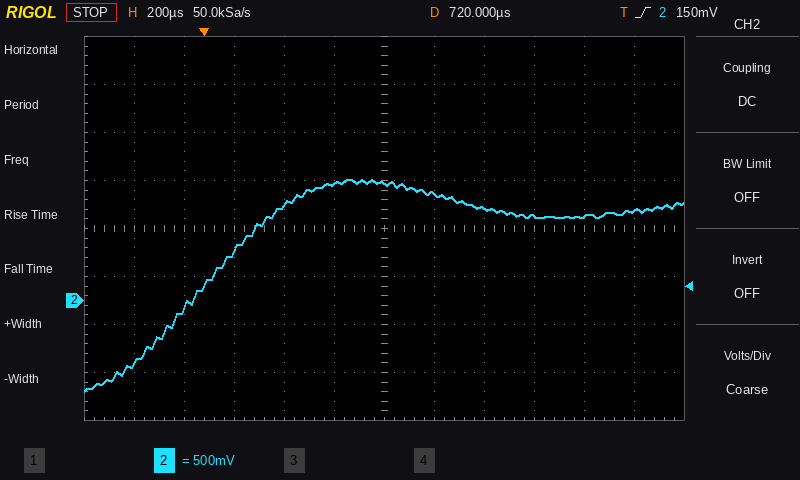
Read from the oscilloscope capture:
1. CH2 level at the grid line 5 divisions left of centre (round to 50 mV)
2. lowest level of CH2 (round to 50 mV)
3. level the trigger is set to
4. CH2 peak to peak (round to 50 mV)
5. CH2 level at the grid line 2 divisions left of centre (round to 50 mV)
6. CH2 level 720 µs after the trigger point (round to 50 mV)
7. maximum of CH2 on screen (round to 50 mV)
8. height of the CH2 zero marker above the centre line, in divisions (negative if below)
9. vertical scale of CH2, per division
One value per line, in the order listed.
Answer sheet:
-650 mV
-950 mV
150 mV
2.20 V
1.00 V
1.20 V
1.25 V
-1.5 div
500 mV
